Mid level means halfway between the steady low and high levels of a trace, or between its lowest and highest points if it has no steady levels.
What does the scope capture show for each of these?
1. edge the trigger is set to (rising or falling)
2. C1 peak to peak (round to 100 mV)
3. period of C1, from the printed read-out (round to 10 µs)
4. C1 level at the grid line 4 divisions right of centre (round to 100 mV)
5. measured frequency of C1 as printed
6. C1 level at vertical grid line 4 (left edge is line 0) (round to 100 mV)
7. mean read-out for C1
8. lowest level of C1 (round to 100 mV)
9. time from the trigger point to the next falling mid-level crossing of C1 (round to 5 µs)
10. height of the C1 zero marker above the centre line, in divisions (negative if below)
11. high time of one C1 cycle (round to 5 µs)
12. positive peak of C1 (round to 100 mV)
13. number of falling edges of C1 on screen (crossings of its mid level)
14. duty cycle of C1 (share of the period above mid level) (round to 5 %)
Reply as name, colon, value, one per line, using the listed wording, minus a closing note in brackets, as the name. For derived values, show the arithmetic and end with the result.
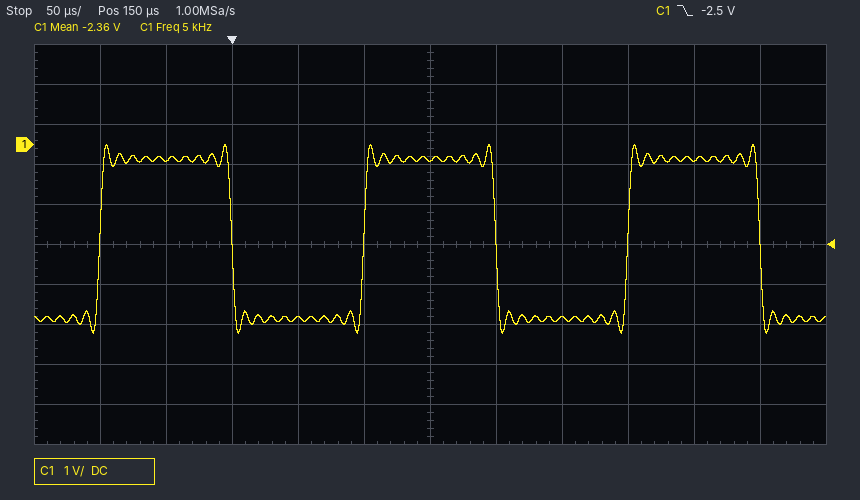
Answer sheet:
edge the trigger is set to: falling
C1 peak to peak: 0.0 V − (-4.7 V) = 4.7 V
period of C1, from the printed read-out: 1 / 5 kHz ≈ 200 µs
C1 level at the grid line 4 divisions right of centre: -400 mV
measured frequency of C1 as printed: 5 kHz
C1 level at vertical grid line 4 (left edge is line 0): -4.3 V
mean read-out for C1: -2.36 V
lowest level of C1: -4.7 V
time from the trigger point to the next falling mid-level crossing of C1: 200 µs
height of the C1 zero marker above the centre line, in divisions: +2.5 div
high time of one C1 cycle: 100 µs
positive peak of C1: 0.0 V
number of falling edges of C1 on screen: 3
duty cycle of C1 (share of the period above mid level): 50 %
